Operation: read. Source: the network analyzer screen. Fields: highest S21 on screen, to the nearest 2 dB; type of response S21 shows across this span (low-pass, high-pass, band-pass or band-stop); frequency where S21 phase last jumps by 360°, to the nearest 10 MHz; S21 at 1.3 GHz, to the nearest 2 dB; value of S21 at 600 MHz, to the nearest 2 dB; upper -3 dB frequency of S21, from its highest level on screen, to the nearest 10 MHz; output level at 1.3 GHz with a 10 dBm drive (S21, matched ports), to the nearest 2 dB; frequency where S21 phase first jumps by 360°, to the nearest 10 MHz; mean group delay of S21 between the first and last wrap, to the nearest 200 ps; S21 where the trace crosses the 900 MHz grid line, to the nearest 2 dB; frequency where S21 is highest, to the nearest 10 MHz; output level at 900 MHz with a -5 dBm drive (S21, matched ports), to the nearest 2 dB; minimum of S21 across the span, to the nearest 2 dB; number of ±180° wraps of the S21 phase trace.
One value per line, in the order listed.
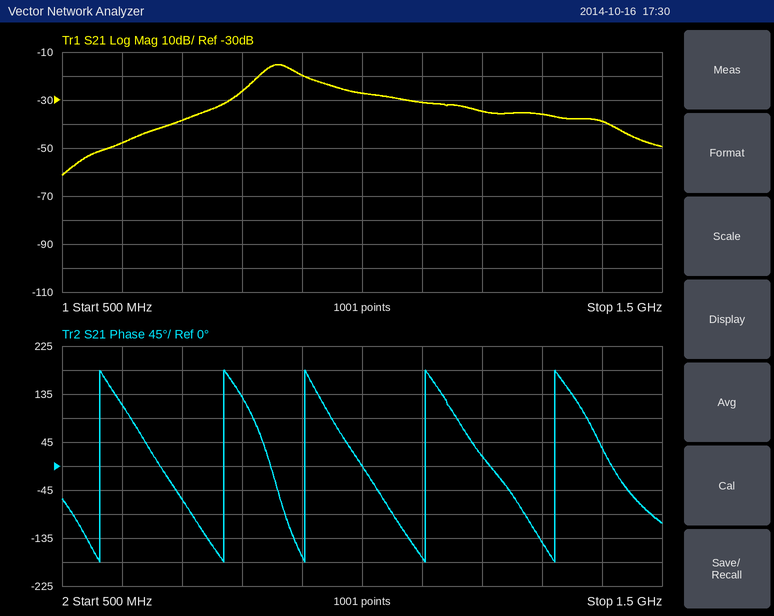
-16 dB
band-pass
1.32 GHz
-36 dB
-48 dB
890 MHz
-26 dBm
560 MHz
5.2 ns
-20 dB
860 MHz
-24 dBm
-62 dB
5
